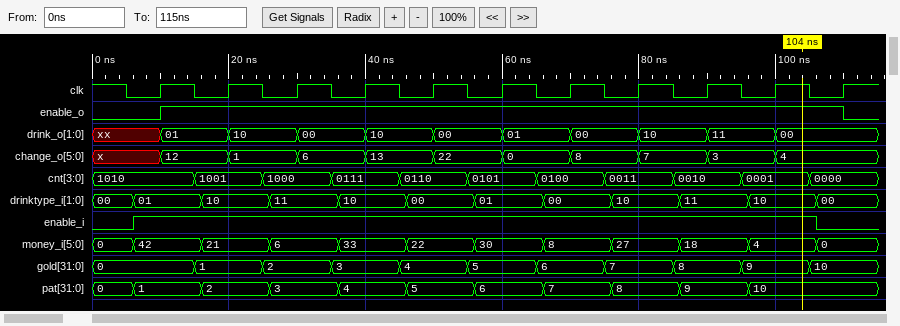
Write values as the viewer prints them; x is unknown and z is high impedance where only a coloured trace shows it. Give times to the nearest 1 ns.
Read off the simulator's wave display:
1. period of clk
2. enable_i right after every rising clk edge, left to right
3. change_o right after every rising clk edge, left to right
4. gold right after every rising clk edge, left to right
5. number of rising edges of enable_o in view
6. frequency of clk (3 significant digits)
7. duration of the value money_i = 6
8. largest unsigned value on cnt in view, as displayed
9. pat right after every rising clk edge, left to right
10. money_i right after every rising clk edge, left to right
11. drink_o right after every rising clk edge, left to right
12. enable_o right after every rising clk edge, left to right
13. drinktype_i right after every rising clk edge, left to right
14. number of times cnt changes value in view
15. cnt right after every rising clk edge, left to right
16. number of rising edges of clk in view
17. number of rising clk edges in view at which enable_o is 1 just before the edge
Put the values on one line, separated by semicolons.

10 ns; 1 1 1 1 1 1 1 1 1 1 0; 12, 1, 6, 13, 22, 0, 8, 7, 3, 4, 4; 0, 1, 2, 3, 4, 5, 6, 7, 8, 9, 10; 1; 100 MHz; 10 ns; 1010; 1, 2, 3, 4, 5, 6, 7, 8, 9, 10, 10; 42, 21, 6, 33, 22, 30, 8, 27, 18, 4, 0; 01, 10, 00, 10, 00, 01, 00, 10, 11, 00, 00; 1 1 1 1 1 1 1 1 1 1 0; 01, 10, 11, 10, 00, 01, 00, 10, 11, 10, 00; 10; 1010, 1001, 1000, 0111, 0110, 0101, 0100, 0011, 0010, 0001, 0000; 11; 10
